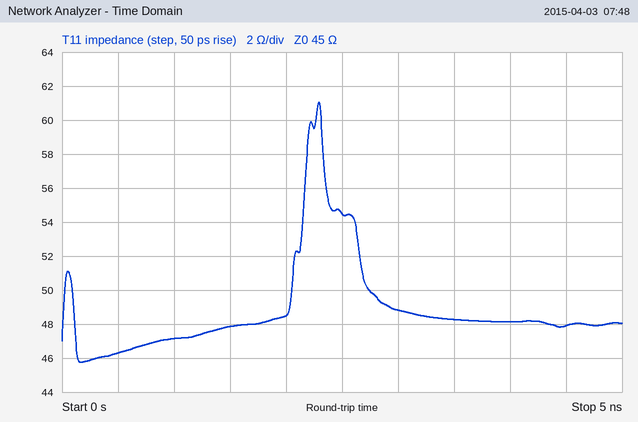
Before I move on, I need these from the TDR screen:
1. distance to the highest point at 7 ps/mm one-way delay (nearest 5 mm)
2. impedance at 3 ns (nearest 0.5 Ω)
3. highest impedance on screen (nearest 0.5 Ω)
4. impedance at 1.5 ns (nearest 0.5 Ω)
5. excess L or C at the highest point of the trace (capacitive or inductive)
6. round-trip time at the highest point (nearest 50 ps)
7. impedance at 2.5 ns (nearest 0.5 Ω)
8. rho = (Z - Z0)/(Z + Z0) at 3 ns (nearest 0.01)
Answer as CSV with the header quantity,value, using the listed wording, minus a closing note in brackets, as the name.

quantity,value
distance to the highest point at 7 ps/mm one-way delay,165 mm
impedance at 3 ns,49.0 Ω
highest impedance on screen,61.0 Ω
impedance at 1.5 ns,48.0 Ω
excess L or C at the highest point of the trace,inductive
round-trip time at the highest point,2.30 ns
impedance at 2.5 ns,54.5 Ω
rho = (Z - Z0)/(Z + Z0) at 3 ns,+0.04
